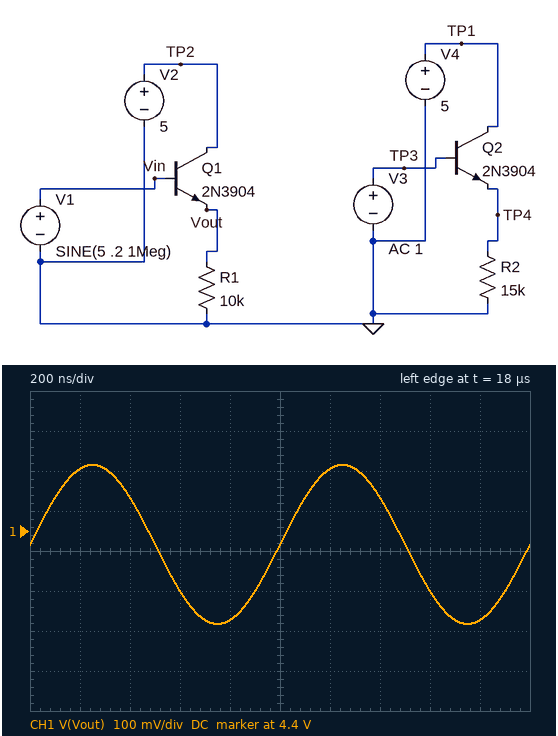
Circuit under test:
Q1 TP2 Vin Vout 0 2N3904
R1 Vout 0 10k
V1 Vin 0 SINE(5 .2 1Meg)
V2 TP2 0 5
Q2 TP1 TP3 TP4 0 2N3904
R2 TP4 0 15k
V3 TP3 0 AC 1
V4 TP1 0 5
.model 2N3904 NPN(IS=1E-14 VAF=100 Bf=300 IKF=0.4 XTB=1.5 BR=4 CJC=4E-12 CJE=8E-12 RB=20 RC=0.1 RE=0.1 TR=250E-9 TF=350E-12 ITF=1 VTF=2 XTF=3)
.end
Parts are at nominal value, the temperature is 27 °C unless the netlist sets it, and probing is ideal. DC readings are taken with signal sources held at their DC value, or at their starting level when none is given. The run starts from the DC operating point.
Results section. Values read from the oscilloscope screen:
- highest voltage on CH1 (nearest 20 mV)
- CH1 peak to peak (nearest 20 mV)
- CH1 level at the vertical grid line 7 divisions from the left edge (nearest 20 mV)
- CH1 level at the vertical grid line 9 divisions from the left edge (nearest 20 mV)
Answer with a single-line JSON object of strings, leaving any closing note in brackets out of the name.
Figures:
{"highest voltage on CH1": "4.56 V", "CH1 peak to peak": "400 mV", "CH1 level at the vertical grid line 7 divisions from the left edge": "4.48 V", "CH1 level at the vertical grid line 9 divisions from the left edge": "4.18 V"}
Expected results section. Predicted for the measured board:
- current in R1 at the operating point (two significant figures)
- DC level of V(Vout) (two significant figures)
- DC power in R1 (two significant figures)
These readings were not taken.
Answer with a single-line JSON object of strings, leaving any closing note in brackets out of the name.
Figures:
{"current in R1 at the operating point": "440 µA", "DC level of V(Vout)": "4.4 V", "DC power in R1": "1.9 mW"}
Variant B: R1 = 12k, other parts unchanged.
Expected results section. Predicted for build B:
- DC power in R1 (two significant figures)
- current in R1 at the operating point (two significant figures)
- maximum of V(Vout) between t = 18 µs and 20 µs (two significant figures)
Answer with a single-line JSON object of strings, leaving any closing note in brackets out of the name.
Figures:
{"DC power in R1": "1.6 mW", "current in R1 at the operating point": "360 µA", "maximum of V(Vout) between t = 18 µs and 20 µs": "4.6 V"}
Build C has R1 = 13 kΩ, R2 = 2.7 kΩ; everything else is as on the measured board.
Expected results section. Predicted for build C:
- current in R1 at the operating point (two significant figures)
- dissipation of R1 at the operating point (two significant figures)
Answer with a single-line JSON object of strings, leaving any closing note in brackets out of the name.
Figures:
{"current in R1 at the operating point": "340 µA", "dissipation of R1 at the operating point": "1.5 mW"}
